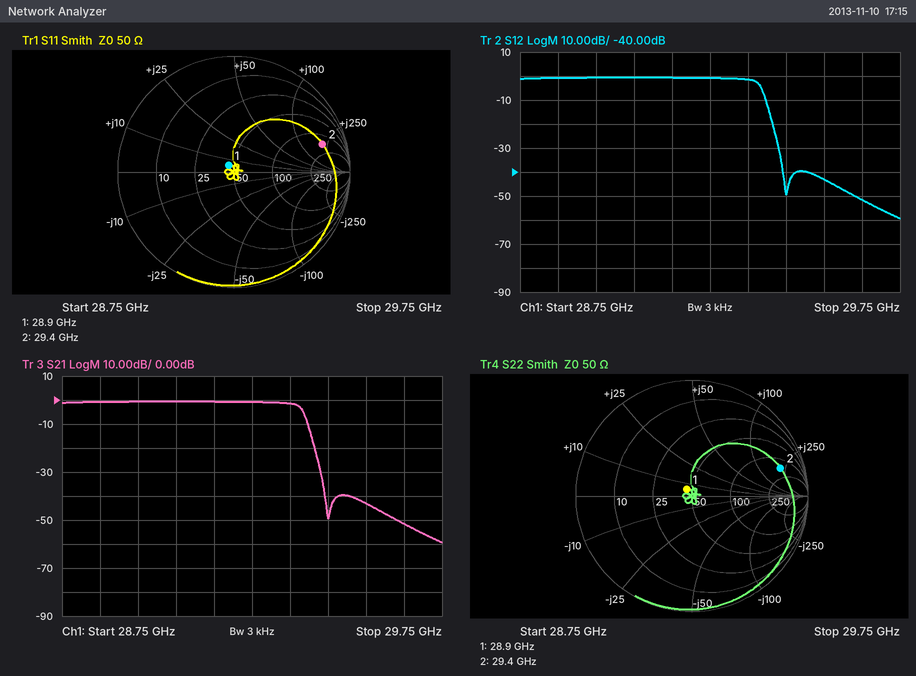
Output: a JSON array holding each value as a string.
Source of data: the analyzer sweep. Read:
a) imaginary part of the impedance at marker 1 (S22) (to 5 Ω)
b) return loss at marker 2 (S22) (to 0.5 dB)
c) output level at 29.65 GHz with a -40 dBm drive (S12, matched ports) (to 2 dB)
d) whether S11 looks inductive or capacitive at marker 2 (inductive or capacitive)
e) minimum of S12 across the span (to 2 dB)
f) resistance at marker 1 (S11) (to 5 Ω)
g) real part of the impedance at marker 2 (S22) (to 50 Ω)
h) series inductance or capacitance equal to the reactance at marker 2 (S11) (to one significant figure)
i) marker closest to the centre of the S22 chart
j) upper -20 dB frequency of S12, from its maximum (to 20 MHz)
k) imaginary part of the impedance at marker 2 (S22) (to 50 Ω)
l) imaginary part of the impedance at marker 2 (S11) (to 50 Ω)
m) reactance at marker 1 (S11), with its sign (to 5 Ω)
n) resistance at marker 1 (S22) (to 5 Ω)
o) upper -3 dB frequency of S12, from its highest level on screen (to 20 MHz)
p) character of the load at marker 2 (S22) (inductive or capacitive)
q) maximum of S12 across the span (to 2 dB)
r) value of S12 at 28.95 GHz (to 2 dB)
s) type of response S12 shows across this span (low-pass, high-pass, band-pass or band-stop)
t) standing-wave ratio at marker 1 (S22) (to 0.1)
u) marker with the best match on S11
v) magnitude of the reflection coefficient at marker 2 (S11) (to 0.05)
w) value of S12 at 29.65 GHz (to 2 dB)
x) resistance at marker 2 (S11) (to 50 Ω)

["+5 Ω", "2.0 dB", "-92 dBm", "inductive", "-60 dB", "45 Ω", "150 Ω", "1 nH", "marker 1", "29.42 GHz", "+200 Ω", "+200 Ω", "+5 Ω", "45 Ω", "29.38 GHz", "inductive", "0 dB", "0 dB", "low-pass", "1.2", "marker 1", "0.80", "-52 dB", "150 Ω"]
